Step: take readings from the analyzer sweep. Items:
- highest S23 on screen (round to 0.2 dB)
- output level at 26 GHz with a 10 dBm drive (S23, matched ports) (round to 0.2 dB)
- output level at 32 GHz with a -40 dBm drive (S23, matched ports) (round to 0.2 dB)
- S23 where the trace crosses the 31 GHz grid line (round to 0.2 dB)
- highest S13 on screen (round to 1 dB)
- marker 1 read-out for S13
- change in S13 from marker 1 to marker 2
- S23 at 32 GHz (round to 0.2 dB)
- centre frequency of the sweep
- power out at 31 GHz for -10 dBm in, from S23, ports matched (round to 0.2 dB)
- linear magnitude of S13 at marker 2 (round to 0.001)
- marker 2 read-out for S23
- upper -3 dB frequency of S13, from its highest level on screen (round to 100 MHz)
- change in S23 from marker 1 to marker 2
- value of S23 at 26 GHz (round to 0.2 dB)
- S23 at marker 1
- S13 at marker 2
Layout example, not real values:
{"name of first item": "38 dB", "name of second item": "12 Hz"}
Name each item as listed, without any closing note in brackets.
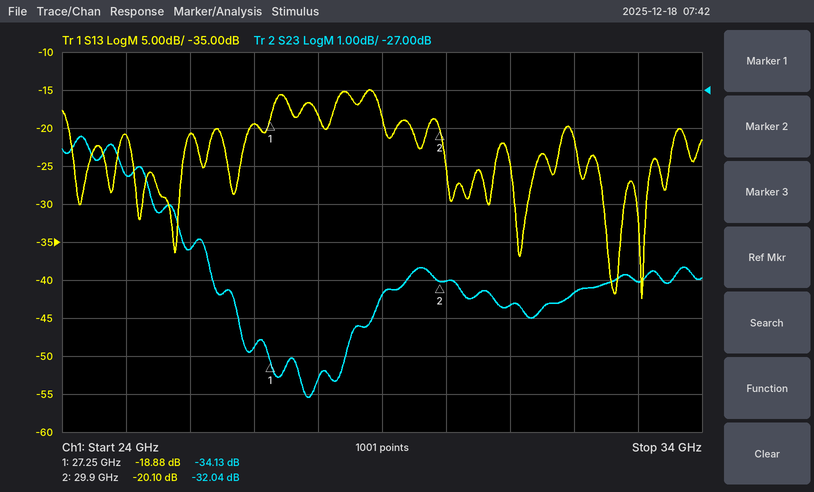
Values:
{"highest S23 on screen": "-28.2 dB", "output level at 26 GHz with a 10 dBm drive (S23, matched ports)": "-21.2 dBm", "output level at 32 GHz with a -40 dBm drive (S23, matched ports)": "-72.4 dBm", "S23 where the trace crosses the 31 GHz grid line": "-32.6 dB", "highest S13 on screen": "-15 dB", "marker 1 read-out for S13": "-18.88 dB", "change in S13 from marker 1 to marker 2": "-1.22 dB", "S23 at 32 GHz": "-32.4 dB", "centre frequency of the sweep": "29 GHz", "power out at 31 GHz for -10 dBm in, from S23, ports matched": "-42.6 dBm", "linear magnitude of S13 at marker 2": "0.099", "marker 2 read-out for S23": "-32.04 dB", "upper -3 dB frequency of S13, from its highest level on screen": "29.0 GHz", "change in S23 from marker 1 to marker 2": "2.09 dB", "value of S23 at 26 GHz": "-31.2 dB", "S23 at marker 1": "-34.13 dB", "S13 at marker 2": "-20.10 dB"}
